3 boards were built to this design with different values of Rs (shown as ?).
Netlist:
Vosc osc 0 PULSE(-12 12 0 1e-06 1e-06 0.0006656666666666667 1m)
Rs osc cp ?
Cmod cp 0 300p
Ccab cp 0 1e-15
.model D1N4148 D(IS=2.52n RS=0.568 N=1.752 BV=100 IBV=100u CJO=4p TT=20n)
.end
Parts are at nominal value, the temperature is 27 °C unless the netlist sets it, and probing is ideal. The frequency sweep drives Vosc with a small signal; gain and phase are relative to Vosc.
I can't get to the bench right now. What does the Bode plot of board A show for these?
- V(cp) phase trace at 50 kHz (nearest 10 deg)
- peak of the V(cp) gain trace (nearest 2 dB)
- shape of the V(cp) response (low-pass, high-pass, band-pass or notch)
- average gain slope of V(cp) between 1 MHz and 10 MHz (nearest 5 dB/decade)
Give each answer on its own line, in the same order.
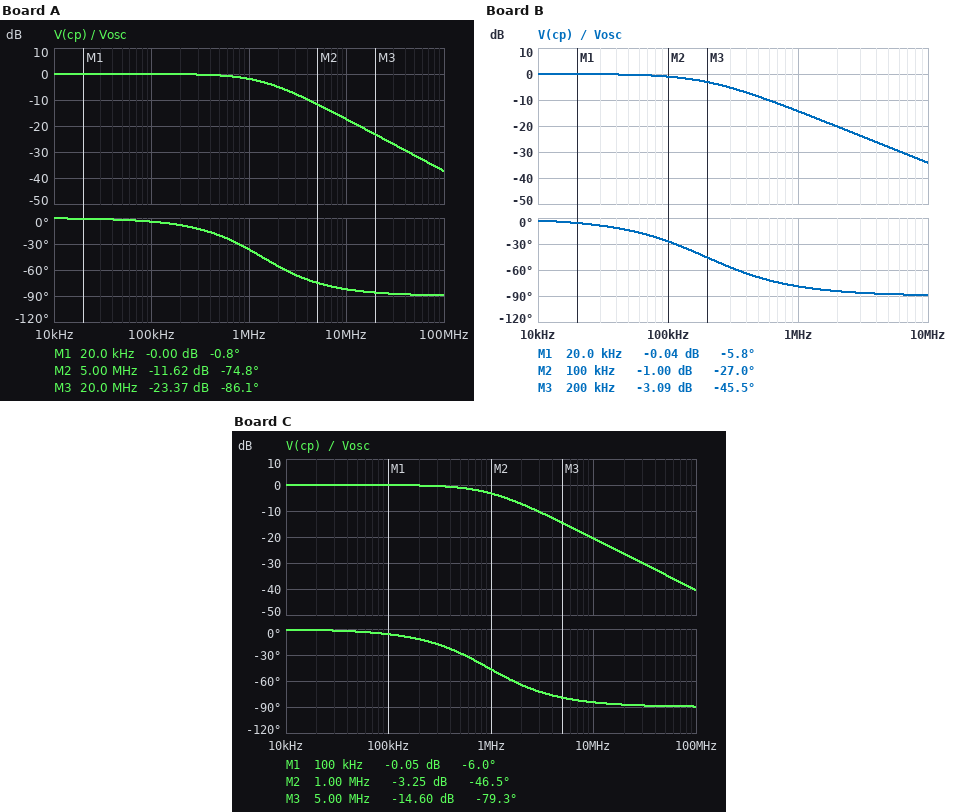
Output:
0 deg
0 dB
low-pass
-15 dB/decade
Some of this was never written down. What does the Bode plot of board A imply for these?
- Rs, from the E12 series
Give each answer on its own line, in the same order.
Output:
390 Ω
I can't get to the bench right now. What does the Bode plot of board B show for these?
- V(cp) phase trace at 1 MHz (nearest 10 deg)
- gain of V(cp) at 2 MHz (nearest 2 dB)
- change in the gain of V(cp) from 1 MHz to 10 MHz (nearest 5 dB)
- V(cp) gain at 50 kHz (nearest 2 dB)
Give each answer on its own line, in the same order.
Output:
-80 deg
-20 dB
-20 dB
0 dB
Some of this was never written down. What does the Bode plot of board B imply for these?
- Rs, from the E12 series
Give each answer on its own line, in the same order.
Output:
2.7 kΩ
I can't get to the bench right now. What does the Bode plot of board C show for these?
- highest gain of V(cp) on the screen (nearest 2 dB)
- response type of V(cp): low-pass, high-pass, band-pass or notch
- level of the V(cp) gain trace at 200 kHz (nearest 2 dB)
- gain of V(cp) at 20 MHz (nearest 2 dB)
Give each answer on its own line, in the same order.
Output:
0 dB
low-pass
0 dB
-26 dB
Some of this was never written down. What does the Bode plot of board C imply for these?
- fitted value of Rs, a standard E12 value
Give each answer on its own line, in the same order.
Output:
560 Ω
